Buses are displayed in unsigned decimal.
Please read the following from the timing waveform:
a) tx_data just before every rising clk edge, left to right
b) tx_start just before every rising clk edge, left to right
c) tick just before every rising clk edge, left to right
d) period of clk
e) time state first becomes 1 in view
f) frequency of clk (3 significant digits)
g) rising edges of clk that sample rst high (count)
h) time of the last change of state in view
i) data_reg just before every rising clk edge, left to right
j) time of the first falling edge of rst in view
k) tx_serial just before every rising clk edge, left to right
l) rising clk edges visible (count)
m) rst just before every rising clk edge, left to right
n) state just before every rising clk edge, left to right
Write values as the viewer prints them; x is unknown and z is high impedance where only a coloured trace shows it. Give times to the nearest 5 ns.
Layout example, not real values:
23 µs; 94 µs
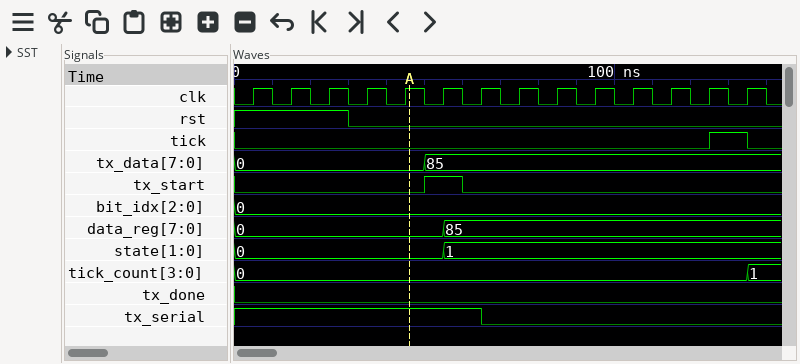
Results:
0, 0, 0, 0, 0, 85, 85, 85, 85, 85, 85, 85, 85, 85; 0 0 0 0 0 1 0 0 0 0 0 0 0 0; 0 0 0 0 0 0 0 0 0 0 0 0 0 1; 10 ns; 55 ns; 100 MHz; 3; 55 ns; 0, 0, 0, 0, 0, 0, 85, 85, 85, 85, 85, 85, 85, 85; 30 ns; 1 1 1 1 1 1 1 0 0 0 0 0 0 0; 14; 1 1 1 0 0 0 0 0 0 0 0 0 0 0; 0, 0, 0, 0, 0, 0, 1, 1, 1, 1, 1, 1, 1, 1
